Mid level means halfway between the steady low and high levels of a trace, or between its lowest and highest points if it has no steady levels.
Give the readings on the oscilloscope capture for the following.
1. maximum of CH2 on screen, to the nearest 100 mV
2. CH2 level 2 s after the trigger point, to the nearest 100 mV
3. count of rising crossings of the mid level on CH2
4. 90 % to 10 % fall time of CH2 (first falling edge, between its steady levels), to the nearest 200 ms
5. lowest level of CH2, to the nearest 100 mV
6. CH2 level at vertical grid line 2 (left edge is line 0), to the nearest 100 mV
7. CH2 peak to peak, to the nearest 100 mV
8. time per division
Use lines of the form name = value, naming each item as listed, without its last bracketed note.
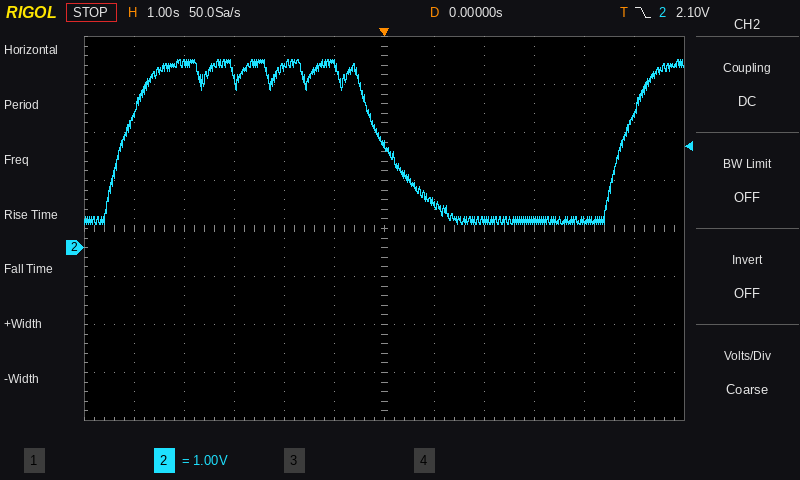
maximum of CH2 on screen, to the nearest 100 mV = 3.9 V
CH2 level 2 s after the trigger point, to the nearest 100 mV = 600 mV
count of rising crossings of the mid level on CH2 = 2
90 % to 10 % fall time of CH2 (first falling edge, between its steady levels), to the nearest 200 ms = 1.6 s
lowest level of CH2, to the nearest 100 mV = 500 mV
CH2 level at vertical grid line 2 (left edge is line 0), to the nearest 100 mV = 3.8 V
CH2 peak to peak, to the nearest 100 mV = 3.4 V
time per division = 1 s
